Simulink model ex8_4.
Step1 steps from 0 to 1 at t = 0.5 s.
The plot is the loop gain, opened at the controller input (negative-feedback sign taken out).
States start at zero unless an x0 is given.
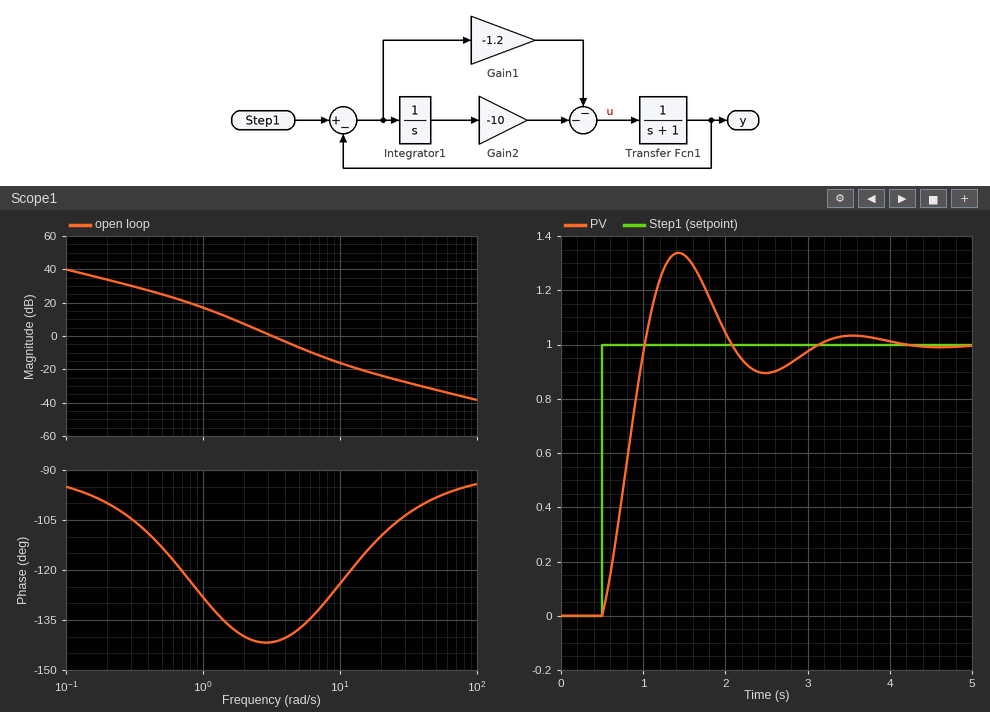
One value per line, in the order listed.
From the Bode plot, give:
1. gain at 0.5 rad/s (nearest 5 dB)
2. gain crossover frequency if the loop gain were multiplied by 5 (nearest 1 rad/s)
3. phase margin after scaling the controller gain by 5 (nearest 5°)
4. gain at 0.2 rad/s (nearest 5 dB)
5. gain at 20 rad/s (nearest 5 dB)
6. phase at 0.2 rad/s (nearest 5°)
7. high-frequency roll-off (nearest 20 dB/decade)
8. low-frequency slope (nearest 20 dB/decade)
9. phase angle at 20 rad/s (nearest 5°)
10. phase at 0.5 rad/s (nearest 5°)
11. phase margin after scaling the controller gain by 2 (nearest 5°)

25 dB
8 rad/s
50°
35 dB
-25 dB
-100°
-20 dB/decade
-20 dB/decade
-110°
-115°
40°
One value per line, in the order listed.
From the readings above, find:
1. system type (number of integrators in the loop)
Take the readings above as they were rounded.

1
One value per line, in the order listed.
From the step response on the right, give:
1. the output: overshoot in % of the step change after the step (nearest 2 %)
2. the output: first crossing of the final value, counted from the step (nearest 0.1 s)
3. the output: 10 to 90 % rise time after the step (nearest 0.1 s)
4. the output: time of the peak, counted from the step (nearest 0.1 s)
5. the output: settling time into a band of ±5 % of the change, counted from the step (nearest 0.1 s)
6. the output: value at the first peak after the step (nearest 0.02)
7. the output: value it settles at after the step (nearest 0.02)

34 %
0.5 s
0.4 s
0.9 s
2.4 s
1.34
1.00
